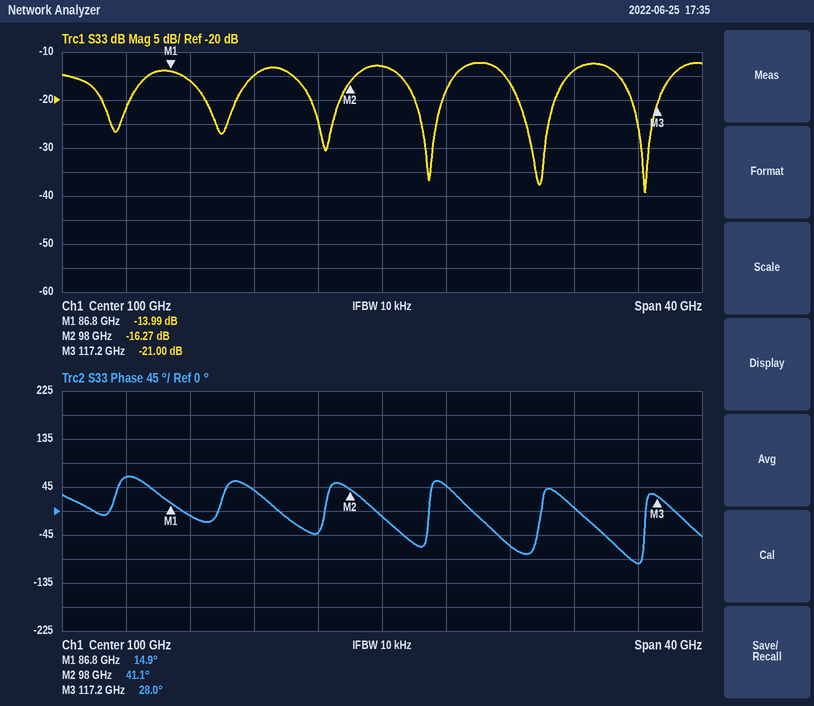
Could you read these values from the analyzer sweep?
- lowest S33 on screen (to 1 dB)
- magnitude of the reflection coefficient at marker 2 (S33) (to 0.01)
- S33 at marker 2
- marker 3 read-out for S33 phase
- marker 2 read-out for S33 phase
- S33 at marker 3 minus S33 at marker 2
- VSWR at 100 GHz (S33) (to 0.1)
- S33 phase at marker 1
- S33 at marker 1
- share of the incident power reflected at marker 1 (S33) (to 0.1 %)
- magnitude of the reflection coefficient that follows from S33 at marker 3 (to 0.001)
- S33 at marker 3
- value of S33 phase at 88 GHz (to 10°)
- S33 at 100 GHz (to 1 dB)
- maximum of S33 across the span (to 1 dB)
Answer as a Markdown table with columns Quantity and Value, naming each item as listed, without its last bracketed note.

| Quantity | Value |
|---|---|
| lowest S33 on screen | -39 dB |
| magnitude of the reflection coefficient at marker 2 (S33) | 0.15 |
| S33 at marker 2 | -16.27 dB |
| marker 3 read-out for S33 phase | 28.0° |
| marker 2 read-out for S33 phase | 41.1° |
| S33 at marker 3 minus S33 at marker 2 | -4.73 dB |
| VSWR at 100 GHz (S33) | 1.6 |
| S33 phase at marker 1 | 14.9° |
| S33 at marker 1 | -13.99 dB |
| share of the incident power reflected at marker 1 (S33) | 4.0 % |
| magnitude of the reflection coefficient that follows from S33 at marker 3 | 0.089 |
| S33 at marker 3 | -21.00 dB |
| value of S33 phase at 88 GHz | -10° |
| S33 at 100 GHz | -13 dB |
| maximum of S33 across the span | -12 dB |
